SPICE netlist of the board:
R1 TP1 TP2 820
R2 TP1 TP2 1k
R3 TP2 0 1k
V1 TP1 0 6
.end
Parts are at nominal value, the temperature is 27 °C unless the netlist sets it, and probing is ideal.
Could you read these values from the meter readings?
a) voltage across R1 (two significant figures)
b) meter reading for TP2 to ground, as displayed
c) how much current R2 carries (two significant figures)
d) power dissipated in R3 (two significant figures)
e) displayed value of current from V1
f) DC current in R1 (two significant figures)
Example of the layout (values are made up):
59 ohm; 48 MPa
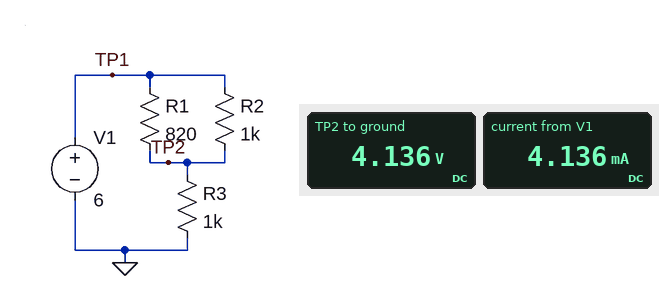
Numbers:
1.9 V; 4.136 V; 1.9 mA; 17 mW; 4.136 mA; 2.3 mA
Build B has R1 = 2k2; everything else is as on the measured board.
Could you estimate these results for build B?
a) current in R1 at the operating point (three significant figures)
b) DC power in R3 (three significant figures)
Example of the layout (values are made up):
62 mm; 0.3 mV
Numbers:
1.11 mA; 12.6 mW
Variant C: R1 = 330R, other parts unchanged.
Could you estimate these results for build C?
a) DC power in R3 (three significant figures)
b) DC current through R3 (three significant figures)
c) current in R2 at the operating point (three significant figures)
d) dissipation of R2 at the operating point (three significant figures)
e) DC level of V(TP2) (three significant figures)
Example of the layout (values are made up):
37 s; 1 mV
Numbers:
23.1 mW; 4.81 mA; 1.19 mA; 1.42 mW; 4.81 V
